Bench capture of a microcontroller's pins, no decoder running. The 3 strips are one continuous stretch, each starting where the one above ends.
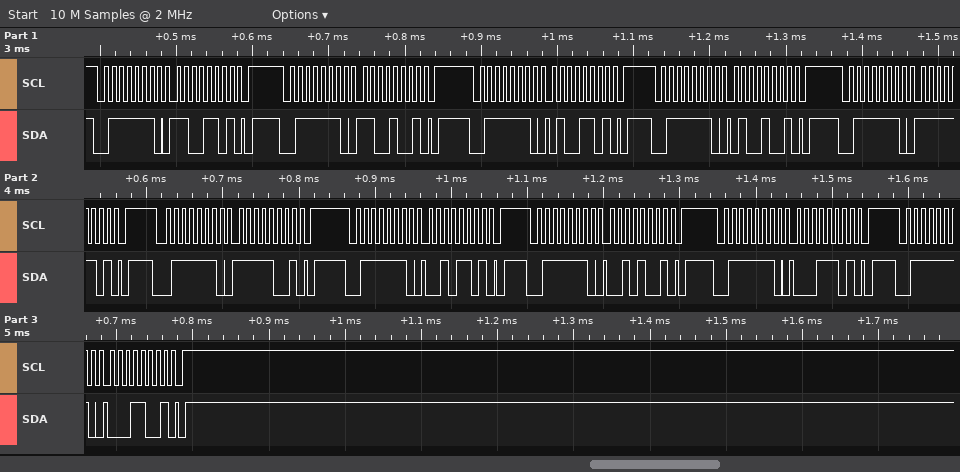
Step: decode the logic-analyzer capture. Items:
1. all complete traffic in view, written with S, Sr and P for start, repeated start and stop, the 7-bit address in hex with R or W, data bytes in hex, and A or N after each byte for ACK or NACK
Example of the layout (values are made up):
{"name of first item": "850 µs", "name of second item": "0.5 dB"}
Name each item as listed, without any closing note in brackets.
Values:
{"all complete traffic in view, written with S, Sr and P for start, repeated start and stop, the 7-bit address in hex with R or W, data bytes in hex, and A or N after each byte for ACK or NACK": "S 3FW A CD A P S 3FW A C9 A P S 3FW A 4D A P S 3FW A 49 A P S 3FW A FD A P S 3FW A F9 A P S 3FW A 2D A P S 3FW A 29 A P S 3FW A 1D A P S 3FW A 19 A P"}
